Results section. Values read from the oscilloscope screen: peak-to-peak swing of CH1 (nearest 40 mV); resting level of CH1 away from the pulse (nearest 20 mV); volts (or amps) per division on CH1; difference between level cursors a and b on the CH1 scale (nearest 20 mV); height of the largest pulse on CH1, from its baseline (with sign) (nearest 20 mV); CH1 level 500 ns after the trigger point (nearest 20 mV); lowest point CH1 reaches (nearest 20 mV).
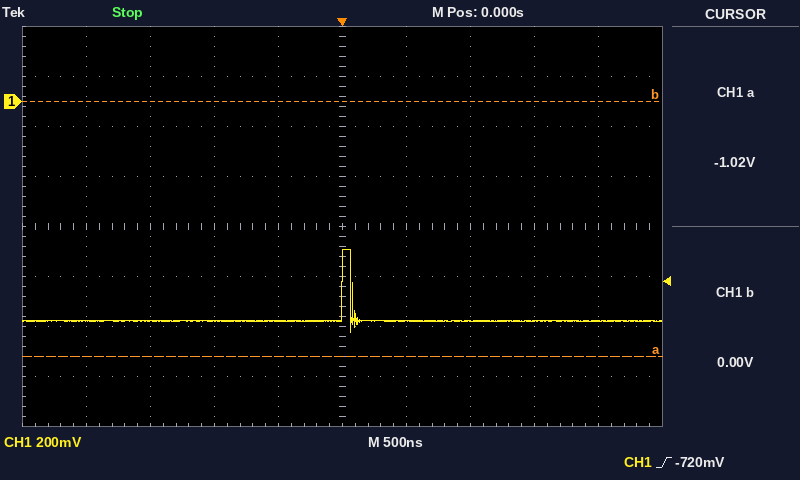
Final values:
320 mV
-880 mV
200 mV
1.02 V
+280 mV
-880 mV
-920 mV
